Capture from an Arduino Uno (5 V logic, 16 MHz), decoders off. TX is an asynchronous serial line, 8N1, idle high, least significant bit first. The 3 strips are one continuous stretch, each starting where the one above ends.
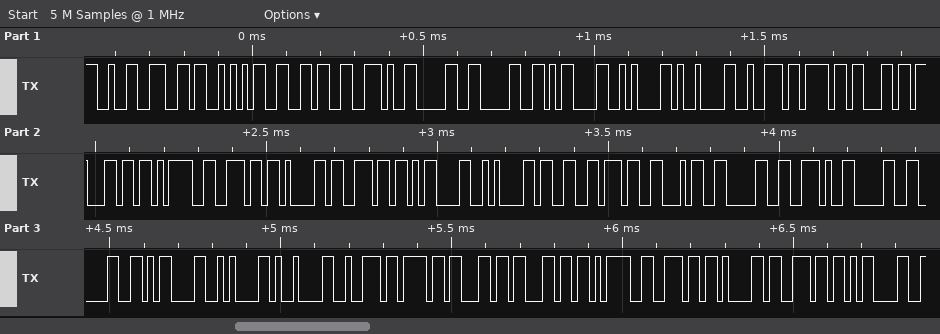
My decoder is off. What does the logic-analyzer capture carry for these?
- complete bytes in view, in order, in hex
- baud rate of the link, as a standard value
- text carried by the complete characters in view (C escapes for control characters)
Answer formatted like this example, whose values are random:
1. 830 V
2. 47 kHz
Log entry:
1. 32 36 35 36 2E 30 30 0D 0A 09 72 6F 6C 6C 3D 6E 61 6E 0D 0A 33 37 34 30 2E 30 30 0D 0A 09 72 6F 6C 6C 3D 6E 61 6E 0D
2. 57600 baud
3. "2656.00\r\n\troll=nan\r\n3740.00\r\n\troll=nan\r"
